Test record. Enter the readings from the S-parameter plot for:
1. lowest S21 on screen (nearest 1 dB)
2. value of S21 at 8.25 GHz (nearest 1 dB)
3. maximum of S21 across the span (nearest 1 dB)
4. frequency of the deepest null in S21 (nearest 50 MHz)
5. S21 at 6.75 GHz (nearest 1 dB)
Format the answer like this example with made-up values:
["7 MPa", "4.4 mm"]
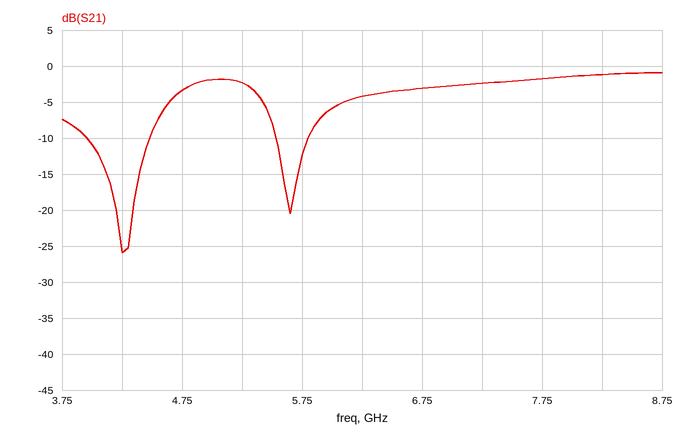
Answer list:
["-26 dB", "-1 dB", "-1 dB", "4.25 GHz", "-3 dB"]
